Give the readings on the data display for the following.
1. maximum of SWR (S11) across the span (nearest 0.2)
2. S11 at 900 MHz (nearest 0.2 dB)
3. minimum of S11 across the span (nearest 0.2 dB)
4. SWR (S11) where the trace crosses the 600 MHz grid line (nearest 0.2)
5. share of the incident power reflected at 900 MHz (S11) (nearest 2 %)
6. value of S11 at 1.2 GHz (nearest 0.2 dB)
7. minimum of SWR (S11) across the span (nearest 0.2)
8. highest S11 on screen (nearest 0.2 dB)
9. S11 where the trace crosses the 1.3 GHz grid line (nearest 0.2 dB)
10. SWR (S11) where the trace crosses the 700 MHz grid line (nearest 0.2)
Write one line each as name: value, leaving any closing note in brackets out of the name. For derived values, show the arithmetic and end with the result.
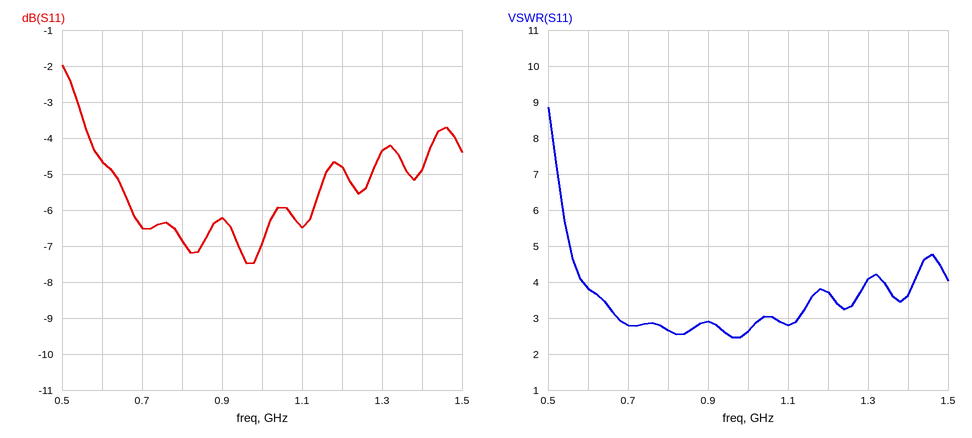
maximum of SWR (S11) across the span: 8.8
S11 at 900 MHz: -6.2 dB
minimum of S11 across the span: -7.4 dB
SWR (S11) where the trace crosses the 600 MHz grid line: 3.8
share of the incident power reflected at 900 MHz (S11): 10^(-6.2/10) ≈ 24 %
value of S11 at 1.2 GHz: -4.8 dB
minimum of SWR (S11) across the span: 2.4
highest S11 on screen: -2.0 dB
S11 where the trace crosses the 1.3 GHz grid line: -4.4 dB
SWR (S11) where the trace crosses the 700 MHz grid line: 2.8
